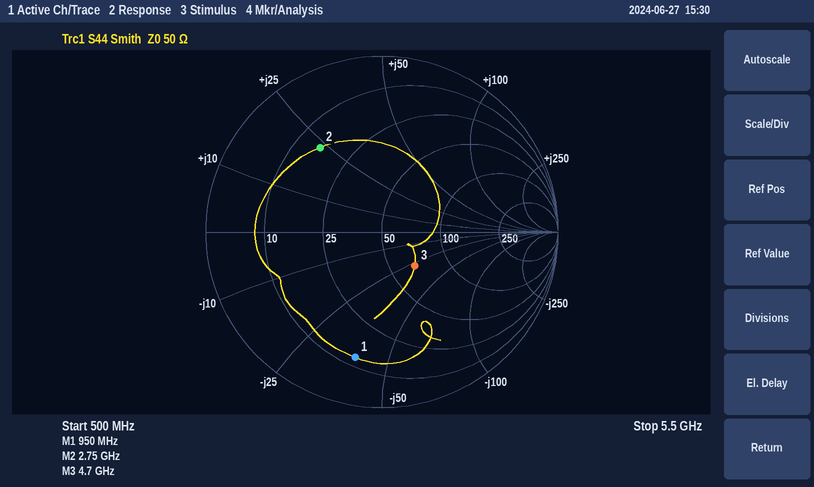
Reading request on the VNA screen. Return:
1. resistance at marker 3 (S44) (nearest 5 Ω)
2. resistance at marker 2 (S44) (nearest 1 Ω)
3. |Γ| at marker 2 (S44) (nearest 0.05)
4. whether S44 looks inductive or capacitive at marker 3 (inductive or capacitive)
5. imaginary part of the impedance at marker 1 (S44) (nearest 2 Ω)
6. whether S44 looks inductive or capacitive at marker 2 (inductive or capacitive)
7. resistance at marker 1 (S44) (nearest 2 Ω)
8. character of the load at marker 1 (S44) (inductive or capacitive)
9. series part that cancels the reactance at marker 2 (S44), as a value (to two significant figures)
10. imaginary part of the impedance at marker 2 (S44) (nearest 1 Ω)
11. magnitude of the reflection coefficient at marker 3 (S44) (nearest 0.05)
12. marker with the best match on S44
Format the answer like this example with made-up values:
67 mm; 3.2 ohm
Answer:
65 Ω; 16 Ω; 0.60; capacitive; -38 Ω; inductive; 12 Ω; capacitive; 2.5 pF; +23 Ω; 0.25; marker 3
